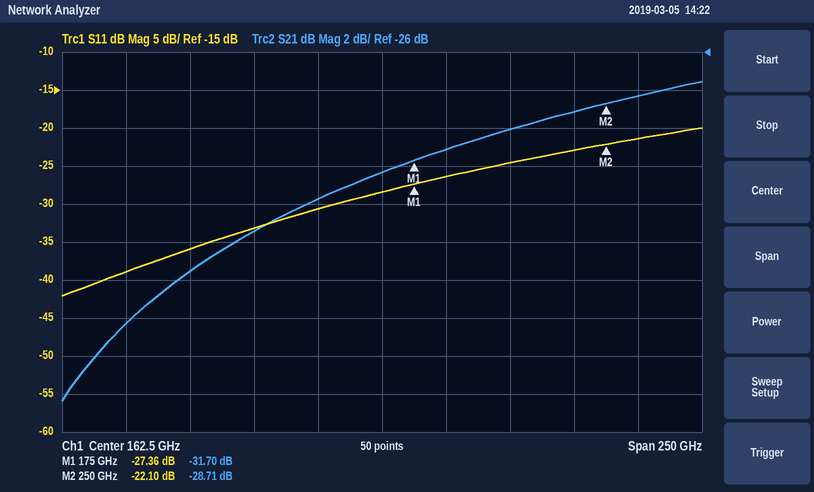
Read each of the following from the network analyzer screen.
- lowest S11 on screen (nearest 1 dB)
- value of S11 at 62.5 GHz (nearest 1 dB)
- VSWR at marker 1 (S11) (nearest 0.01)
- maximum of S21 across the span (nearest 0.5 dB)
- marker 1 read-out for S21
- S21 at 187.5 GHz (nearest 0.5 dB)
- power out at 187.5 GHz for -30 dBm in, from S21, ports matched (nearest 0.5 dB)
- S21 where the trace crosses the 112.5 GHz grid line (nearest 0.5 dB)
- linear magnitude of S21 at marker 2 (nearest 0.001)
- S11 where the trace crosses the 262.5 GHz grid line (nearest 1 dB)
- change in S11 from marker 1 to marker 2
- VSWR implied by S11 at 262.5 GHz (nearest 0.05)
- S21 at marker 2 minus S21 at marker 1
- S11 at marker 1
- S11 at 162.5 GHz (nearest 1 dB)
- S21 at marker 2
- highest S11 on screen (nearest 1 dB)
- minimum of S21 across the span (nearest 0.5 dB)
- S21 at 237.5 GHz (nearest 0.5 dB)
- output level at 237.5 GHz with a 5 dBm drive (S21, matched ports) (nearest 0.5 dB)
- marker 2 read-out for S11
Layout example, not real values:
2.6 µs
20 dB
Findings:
-42 dB
-39 dB
1.09
-27.5 dB
-31.70 dB
-31.0 dB
-61.0 dBm
-35.5 dB
0.037
-21 dB
5.26 dB
1.20
2.99 dB
-27.36 dB
-28 dB
-28.71 dB
-20 dB
-44.5 dB
-29.0 dB
-24.0 dBm
-22.10 dB
